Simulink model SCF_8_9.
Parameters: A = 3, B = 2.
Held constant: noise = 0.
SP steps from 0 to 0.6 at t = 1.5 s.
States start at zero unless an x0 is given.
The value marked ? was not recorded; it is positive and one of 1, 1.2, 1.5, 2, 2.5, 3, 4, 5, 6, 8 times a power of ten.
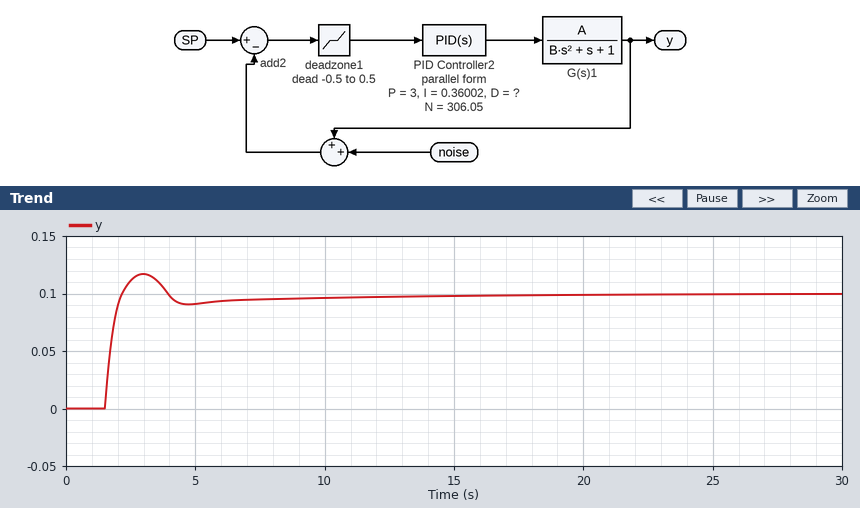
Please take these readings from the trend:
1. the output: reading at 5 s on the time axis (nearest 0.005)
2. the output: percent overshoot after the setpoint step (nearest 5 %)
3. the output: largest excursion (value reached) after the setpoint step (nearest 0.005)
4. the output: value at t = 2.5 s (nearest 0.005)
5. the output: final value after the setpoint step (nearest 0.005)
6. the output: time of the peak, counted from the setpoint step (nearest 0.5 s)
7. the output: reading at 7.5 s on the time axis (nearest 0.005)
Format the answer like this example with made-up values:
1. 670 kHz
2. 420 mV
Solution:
1. 0.090
2. 15 %
3. 0.115
4. 0.110
5. 0.100
6. 1.5 s
7. 0.095
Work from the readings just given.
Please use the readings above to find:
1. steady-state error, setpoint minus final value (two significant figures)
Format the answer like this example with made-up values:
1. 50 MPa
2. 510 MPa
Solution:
1. 0.50
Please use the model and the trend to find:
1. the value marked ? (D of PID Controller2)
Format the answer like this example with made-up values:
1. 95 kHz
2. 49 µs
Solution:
1. 2
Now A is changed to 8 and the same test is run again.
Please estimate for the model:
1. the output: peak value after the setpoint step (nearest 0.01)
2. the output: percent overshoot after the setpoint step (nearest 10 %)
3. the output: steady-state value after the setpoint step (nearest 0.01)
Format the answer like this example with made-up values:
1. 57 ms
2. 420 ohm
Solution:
1. 0.13
2. 30 %
3. 0.10
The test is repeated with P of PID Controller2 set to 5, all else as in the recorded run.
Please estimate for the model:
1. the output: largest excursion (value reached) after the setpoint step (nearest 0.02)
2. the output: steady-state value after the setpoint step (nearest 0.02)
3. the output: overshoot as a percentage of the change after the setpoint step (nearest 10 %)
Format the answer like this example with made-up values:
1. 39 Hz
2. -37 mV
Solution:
1. 0.16
2. 0.10
3. 50 %
